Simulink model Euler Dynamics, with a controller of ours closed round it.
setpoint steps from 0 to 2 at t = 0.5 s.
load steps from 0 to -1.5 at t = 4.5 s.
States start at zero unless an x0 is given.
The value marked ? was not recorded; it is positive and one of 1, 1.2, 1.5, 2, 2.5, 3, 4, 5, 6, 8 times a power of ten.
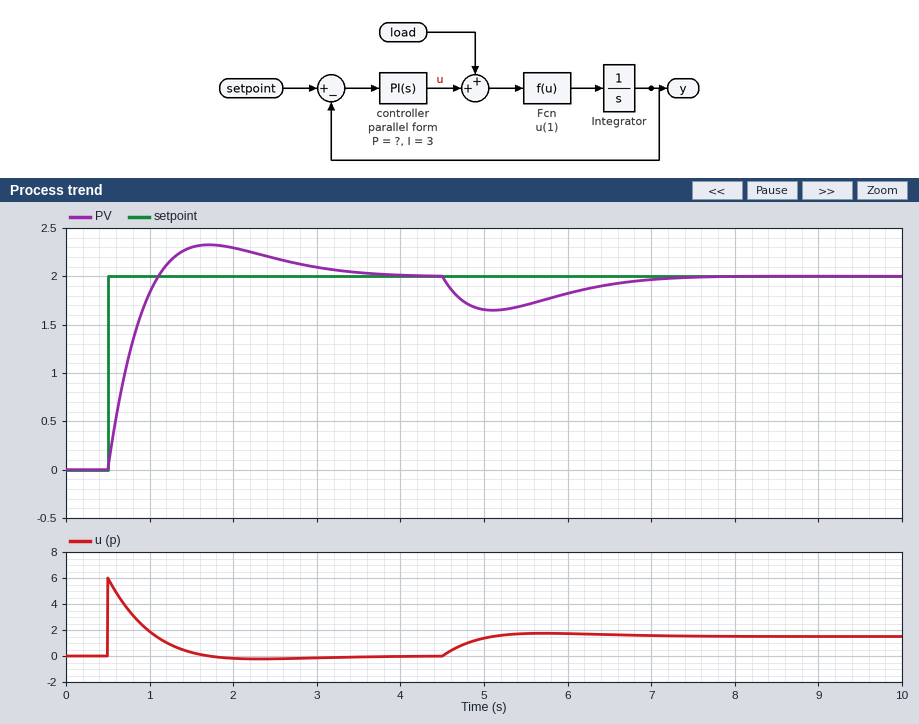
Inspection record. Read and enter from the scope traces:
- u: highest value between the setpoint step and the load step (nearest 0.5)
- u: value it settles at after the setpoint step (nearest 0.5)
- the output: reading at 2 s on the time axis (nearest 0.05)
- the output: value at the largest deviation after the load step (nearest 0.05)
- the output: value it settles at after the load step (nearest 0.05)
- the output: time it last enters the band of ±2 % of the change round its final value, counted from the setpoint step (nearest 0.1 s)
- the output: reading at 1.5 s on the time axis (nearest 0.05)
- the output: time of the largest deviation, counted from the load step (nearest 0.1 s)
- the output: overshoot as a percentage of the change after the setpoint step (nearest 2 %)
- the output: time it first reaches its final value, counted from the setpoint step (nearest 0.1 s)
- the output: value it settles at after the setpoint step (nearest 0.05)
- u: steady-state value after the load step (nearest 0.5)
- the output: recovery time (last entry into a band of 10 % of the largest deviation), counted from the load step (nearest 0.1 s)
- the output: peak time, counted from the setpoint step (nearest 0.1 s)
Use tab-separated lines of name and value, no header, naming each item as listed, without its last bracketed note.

u: highest value between the setpoint step and the load step	6.0
u: value it settles at after the setpoint step	0.0
the output: reading at 2 s on the time axis	2.30
the output: value at the largest deviation after the load step	1.65
the output: value it settles at after the load step	2.00
the output: time it last enters the band of ±2 % of the change round its final value, counted from the setpoint step	3.0 s
the output: reading at 1.5 s on the time axis	2.30
the output: time of the largest deviation, counted from the load step	0.6 s
the output: overshoot as a percentage of the change after the setpoint step	16 %
the output: time it first reaches its final value, counted from the setpoint step	0.6 s
the output: value it settles at after the setpoint step	2.00
u: steady-state value after the load step	1.5
the output: recovery time (last entry into a band of 10 % of the largest deviation), counted from the load step	2.5 s
the output: peak time, counted from the setpoint step	1.2 s
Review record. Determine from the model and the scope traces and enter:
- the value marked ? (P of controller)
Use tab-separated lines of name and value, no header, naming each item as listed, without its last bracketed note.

the value marked ?	3
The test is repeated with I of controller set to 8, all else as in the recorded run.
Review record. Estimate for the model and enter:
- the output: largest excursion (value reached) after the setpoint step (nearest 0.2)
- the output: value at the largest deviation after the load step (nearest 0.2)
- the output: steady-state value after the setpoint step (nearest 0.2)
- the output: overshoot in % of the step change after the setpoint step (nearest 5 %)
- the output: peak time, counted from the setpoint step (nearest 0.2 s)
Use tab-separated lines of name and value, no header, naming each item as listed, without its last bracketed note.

the output: largest excursion (value reached) after the setpoint step	2.6
the output: value at the largest deviation after the load step	1.8
the output: steady-state value after the setpoint step	2.0
the output: overshoot in % of the step change after the setpoint step	30 %
the output: peak time, counted from the setpoint step	0.8 s
